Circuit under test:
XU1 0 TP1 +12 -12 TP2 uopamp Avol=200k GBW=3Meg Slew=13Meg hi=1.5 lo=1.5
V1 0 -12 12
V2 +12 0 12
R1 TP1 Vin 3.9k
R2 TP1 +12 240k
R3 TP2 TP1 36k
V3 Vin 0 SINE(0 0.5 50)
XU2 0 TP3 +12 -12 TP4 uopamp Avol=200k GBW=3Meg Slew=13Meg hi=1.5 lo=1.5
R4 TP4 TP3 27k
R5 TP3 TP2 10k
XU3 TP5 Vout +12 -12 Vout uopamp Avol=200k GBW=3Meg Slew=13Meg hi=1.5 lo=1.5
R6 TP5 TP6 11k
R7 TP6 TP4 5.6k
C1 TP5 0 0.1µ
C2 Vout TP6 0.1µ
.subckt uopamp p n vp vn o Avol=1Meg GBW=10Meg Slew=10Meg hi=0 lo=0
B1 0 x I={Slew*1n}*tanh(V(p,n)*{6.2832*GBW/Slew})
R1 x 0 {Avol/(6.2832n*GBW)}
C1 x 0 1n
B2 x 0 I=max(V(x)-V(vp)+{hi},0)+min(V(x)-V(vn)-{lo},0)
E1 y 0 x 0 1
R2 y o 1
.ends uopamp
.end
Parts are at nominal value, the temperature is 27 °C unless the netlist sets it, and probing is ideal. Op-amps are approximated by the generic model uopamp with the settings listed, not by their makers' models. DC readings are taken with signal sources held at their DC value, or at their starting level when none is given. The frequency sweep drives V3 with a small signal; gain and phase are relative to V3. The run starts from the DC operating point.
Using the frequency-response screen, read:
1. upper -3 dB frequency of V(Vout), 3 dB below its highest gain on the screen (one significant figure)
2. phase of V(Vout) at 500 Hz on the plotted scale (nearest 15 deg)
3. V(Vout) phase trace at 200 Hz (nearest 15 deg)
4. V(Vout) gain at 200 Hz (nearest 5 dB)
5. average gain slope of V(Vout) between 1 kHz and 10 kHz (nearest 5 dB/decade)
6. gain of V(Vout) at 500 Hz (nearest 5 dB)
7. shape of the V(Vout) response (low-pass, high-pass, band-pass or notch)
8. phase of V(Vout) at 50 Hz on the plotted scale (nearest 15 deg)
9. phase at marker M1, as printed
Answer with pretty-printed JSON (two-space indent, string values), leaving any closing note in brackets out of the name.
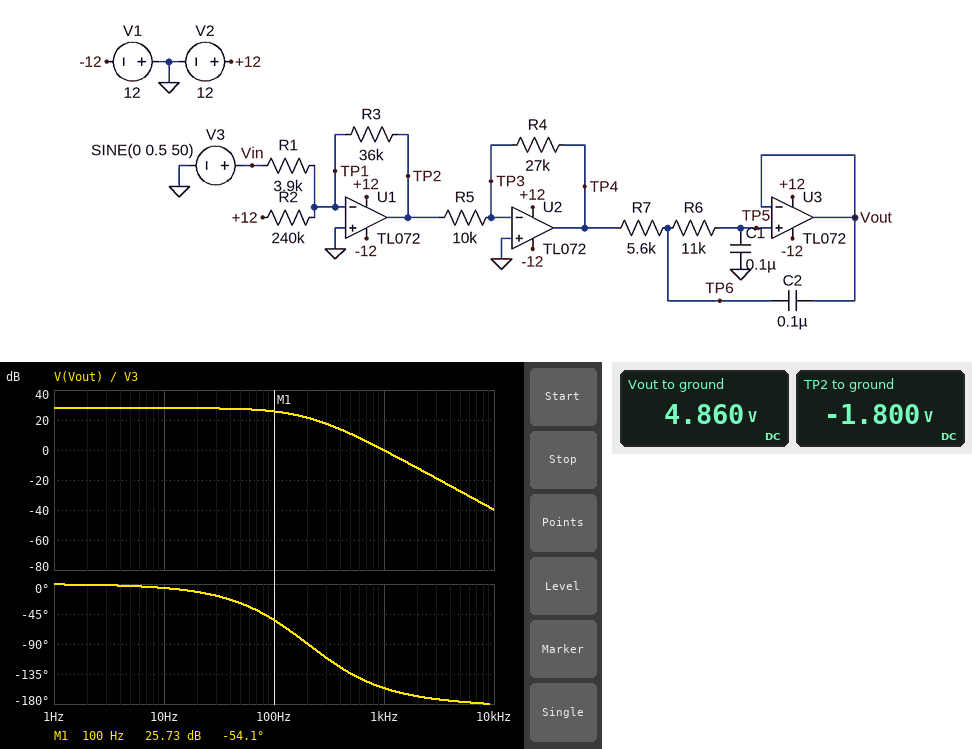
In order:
{
  "upper -3 dB frequency of V(Vout), 3 dB below its highest gain on the screen": "100 Hz",
  "phase of V(Vout) at 500 Hz on the plotted scale": "-135 deg",
  "V(Vout) phase trace at 200 Hz": "-90 deg",
  "V(Vout) gain at 200 Hz": "20 dB",
  "average gain slope of V(Vout) between 1 kHz and 10 kHz": "-40 dB/decade",
  "gain of V(Vout) at 500 Hz": "10 dB",
  "shape of the V(Vout) response": "low-pass",
  "phase of V(Vout) at 50 Hz on the plotted scale": "-30 deg",
  "phase at marker M1, as printed": "-54.1 deg"
}
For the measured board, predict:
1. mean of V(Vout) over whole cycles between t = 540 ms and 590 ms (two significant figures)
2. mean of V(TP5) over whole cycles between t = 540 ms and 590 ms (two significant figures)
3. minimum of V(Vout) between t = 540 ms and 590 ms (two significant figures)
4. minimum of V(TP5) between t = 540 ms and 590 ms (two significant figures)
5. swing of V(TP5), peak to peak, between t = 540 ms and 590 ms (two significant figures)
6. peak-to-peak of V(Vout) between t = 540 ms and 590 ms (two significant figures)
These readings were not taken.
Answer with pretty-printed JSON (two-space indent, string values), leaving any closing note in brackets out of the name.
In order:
{
  "mean of V(Vout) over whole cycles between t = 540 ms and 590 ms": "3.3 V",
  "mean of V(TP5) over whole cycles between t = 540 ms and 590 ms": "3.3 V",
  "minimum of V(Vout) between t = 540 ms and 590 ms": "-6.7 V",
  "minimum of V(TP5) between t = 540 ms and 590 ms": "-6.7 V",
  "swing of V(TP5), peak to peak, between t = 540 ms and 590 ms": "17 V",
  "peak-to-peak of V(Vout) between t = 540 ms and 590 ms": "17 V"
}
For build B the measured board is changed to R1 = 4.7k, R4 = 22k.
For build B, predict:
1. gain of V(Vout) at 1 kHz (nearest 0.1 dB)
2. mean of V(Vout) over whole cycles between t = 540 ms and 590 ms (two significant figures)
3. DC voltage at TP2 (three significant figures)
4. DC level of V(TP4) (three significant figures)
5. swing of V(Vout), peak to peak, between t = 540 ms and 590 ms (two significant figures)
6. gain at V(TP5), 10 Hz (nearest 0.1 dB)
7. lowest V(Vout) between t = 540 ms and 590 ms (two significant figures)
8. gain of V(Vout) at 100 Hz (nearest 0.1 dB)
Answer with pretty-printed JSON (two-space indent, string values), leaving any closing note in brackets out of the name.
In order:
{
  "gain of V(Vout) at 1 kHz": "-3.6 dB",
  "mean of V(Vout) over whole cycles between t = 540 ms and 590 ms": "3.7 V",
  "DC voltage at TP2": "-1.80 V",
  "DC level of V(TP4)": "3.96 V",
  "swing of V(Vout), peak to peak, between t = 540 ms and 590 ms": "14 V",
  "gain at V(TP5), 10 Hz": "24.5 dB",
  "lowest V(Vout) between t = 540 ms and 590 ms": "-3.9 V",
  "gain of V(Vout) at 100 Hz": "22.3 dB"
}
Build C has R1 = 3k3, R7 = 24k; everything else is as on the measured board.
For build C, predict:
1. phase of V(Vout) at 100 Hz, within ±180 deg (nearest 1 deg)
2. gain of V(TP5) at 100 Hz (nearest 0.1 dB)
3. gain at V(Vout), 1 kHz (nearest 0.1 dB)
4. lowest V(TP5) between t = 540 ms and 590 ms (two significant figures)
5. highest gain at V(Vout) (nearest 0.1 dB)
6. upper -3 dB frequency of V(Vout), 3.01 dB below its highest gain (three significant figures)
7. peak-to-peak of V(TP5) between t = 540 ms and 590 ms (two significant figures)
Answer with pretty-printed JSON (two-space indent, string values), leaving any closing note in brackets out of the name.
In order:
{
  "phase of V(Vout) at 100 Hz, within ±180 deg": "-91 deg",
  "gain of V(TP5) at 100 Hz": "22.5 dB",
  "gain at V(Vout), 1 kHz": "-11.1 dB",
  "lowest V(TP5) between t = 540 ms and 590 ms": "-6.4 V",
  "highest gain at V(Vout)": "29.4 dB",
  "upper -3 dB frequency of V(Vout), 3.01 dB below its highest gain": "56.8 Hz",
  "peak-to-peak of V(TP5) between t = 540 ms and 590 ms": "16 V"
}
